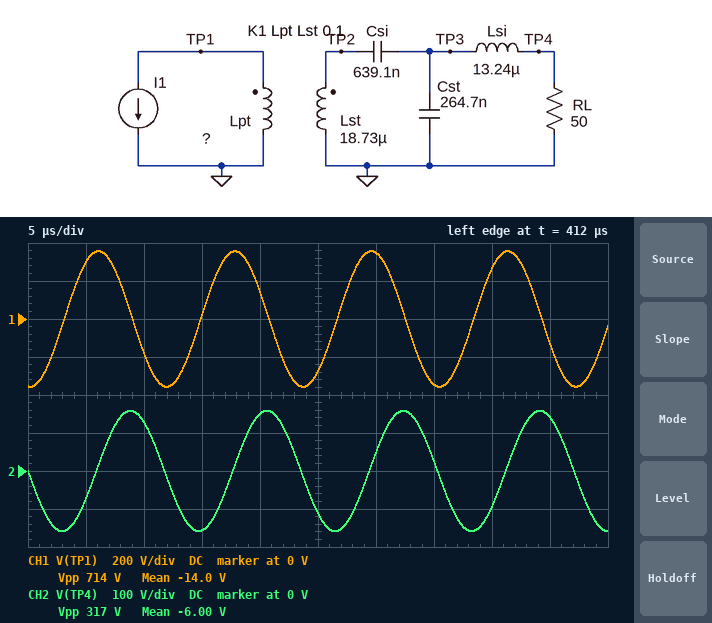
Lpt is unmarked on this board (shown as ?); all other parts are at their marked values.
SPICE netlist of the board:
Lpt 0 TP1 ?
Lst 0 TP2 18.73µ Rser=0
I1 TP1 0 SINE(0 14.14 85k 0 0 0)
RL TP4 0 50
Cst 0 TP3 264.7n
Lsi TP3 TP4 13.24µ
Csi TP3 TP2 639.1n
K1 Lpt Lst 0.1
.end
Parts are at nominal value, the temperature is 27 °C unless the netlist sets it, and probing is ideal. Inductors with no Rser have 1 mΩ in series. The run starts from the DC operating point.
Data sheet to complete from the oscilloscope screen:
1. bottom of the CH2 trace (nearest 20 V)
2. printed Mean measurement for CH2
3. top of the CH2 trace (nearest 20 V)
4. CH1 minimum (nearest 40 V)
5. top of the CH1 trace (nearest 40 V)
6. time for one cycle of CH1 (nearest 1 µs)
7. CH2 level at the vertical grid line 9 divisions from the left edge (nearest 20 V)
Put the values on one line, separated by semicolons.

-160 V; -6.00 V; 160 V; -360 V; 360 V; 12 µs; 140 V
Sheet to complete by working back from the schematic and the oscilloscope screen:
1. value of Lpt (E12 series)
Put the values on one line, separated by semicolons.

47 µH
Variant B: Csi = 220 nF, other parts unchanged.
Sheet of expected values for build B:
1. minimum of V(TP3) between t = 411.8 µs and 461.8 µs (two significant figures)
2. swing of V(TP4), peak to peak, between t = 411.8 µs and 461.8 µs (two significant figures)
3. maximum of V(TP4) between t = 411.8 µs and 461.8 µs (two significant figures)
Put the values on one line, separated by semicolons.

-28 V; 56 V; 28 V
